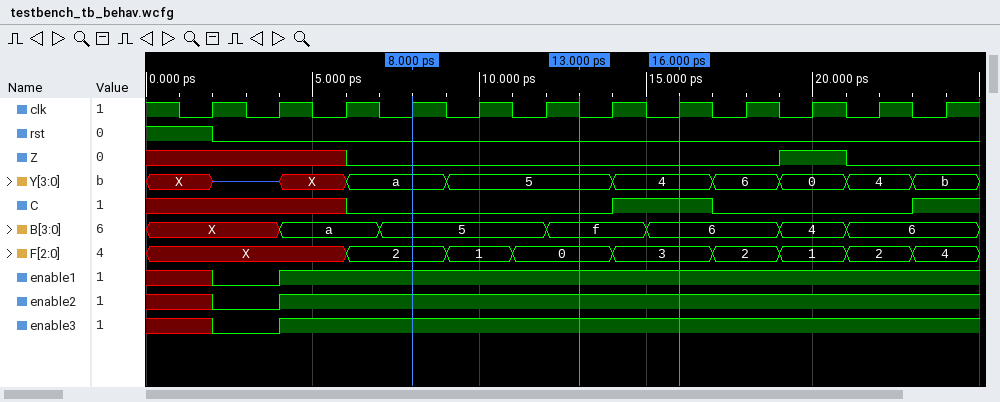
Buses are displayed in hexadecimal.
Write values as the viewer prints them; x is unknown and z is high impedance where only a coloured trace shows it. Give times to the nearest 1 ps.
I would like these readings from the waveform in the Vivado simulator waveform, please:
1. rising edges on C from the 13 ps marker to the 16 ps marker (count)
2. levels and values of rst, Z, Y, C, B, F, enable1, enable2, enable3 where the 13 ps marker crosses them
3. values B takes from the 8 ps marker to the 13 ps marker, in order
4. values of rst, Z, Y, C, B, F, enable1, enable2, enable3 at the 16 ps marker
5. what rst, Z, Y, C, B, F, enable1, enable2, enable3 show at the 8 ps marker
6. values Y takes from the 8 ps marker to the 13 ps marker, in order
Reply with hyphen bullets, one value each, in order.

- 1
- rst=0, Z=0, Y=5, C=0, B=f, F=0, enable1=1, enable2=1, enable3=1
- 5, f
- rst=0, Z=0, Y=4, C=1, B=6, F=3, enable1=1, enable2=1, enable3=1
- rst=0, Z=0, Y=a, C=0, B=5, F=2, enable1=1, enable2=1, enable3=1
- a, 5
